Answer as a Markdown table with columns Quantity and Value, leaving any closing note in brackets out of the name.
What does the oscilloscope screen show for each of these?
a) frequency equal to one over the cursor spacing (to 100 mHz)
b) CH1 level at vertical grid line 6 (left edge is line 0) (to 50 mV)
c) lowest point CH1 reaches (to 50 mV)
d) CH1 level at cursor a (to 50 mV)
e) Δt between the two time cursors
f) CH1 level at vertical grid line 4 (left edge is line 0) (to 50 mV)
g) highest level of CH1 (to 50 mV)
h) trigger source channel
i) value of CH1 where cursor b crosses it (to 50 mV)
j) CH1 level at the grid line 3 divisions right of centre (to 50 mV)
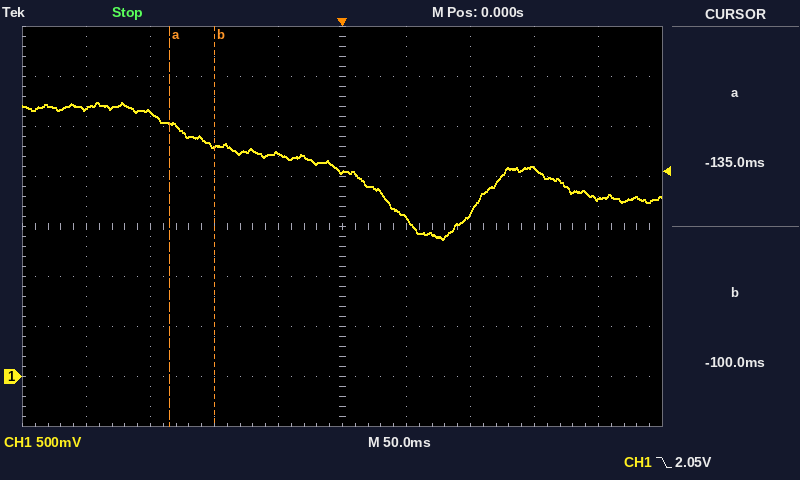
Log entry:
| Quantity | Value |
|---|---|
| frequency equal to one over the cursor spacing | 28.6 Hz |
| CH1 level at vertical grid line 6 (left edge is line 0) | 1.60 V |
| lowest point CH1 reaches | 1.35 V |
| CH1 level at cursor a | 2.55 V |
| Δt between the two time cursors | 35 ms |
| CH1 level at vertical grid line 4 (left edge is line 0) | 2.25 V |
| highest level of CH1 | 2.75 V |
| trigger source channel | CH1 |
| value of CH1 where cursor b crosses it | 2.30 V |
| CH1 level at the grid line 3 divisions right of centre | 2.10 V |
